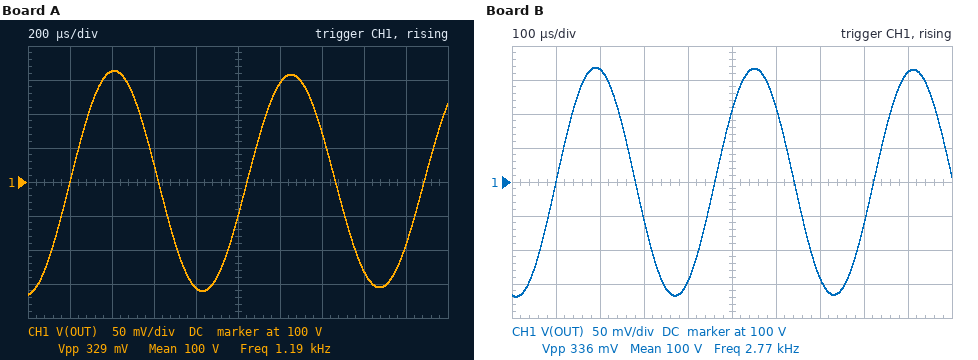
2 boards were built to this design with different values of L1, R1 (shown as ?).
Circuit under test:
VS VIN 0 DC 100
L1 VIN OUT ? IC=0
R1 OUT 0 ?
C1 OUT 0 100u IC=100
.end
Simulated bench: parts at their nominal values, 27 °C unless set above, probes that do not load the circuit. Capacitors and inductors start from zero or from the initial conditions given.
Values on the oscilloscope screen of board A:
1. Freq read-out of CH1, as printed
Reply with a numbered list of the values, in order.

1. 1.19 kHz
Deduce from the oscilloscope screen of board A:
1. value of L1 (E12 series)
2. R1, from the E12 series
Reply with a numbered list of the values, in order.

1. 180 µH
2. 120 Ω
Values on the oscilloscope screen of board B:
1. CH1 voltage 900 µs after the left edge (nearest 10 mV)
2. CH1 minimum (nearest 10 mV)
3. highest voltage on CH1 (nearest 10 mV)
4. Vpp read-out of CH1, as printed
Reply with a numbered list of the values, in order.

1. 100.16 V
2. 99.83 V
3. 100.17 V
4. 336 mV
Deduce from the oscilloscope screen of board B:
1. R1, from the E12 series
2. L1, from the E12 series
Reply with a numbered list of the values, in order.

1. 220 Ω
2. 33 µH
